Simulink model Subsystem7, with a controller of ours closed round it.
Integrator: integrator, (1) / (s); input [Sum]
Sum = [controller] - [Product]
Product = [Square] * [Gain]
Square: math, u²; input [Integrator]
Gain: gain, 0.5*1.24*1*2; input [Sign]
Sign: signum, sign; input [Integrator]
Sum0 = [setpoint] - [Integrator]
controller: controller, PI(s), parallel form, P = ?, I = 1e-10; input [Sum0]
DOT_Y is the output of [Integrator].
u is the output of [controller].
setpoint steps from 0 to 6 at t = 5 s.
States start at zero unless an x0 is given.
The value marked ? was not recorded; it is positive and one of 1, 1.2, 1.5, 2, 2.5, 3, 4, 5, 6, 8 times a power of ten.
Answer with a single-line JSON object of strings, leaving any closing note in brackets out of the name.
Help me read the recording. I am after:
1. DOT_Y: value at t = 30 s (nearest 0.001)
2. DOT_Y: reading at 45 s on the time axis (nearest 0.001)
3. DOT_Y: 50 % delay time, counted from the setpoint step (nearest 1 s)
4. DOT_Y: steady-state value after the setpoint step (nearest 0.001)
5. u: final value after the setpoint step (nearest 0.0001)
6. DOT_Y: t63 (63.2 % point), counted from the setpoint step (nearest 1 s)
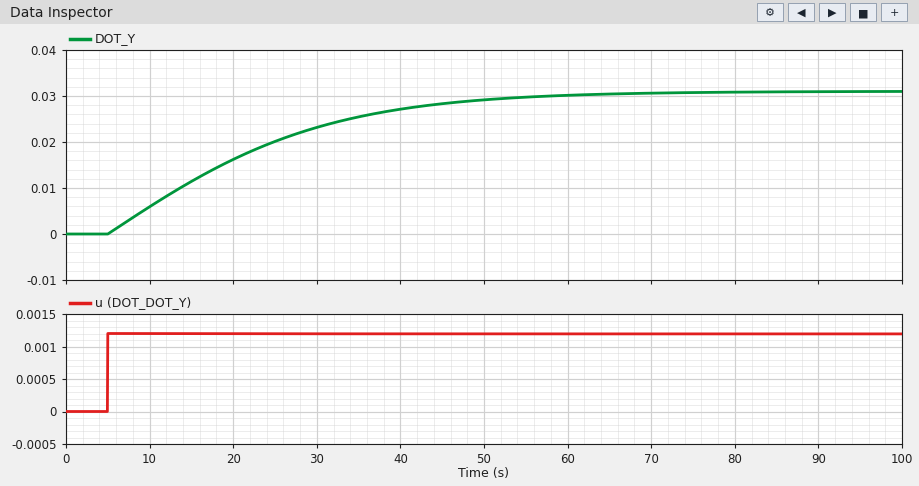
{"DOT_Y: value at t = 30 s": "0.023", "DOT_Y: reading at 45 s on the time axis": "0.028", "DOT_Y: 50 % delay time, counted from the setpoint step": "14 s", "DOT_Y: steady-state value after the setpoint step": "0.031", "u: final value after the setpoint step": "0.0012", "DOT_Y: t63 (63.2 % point), counted from the setpoint step": "19 s"}
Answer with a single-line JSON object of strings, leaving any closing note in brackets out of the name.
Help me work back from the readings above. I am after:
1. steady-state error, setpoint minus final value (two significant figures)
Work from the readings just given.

{"steady-state error, setpoint minus final value": "6.0"}
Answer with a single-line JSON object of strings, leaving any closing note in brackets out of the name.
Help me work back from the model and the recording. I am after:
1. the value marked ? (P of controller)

{"the value marked ?": "0.0002"}
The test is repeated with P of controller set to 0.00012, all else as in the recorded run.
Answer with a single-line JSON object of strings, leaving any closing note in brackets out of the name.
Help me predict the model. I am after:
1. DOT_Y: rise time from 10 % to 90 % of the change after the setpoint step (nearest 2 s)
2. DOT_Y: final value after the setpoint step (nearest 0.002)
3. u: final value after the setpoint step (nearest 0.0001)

{"DOT_Y: rise time from 10 % to 90 % of the change after the setpoint step": "46 s", "DOT_Y: final value after the setpoint step": "0.024", "u: final value after the setpoint step": "0.0007"}
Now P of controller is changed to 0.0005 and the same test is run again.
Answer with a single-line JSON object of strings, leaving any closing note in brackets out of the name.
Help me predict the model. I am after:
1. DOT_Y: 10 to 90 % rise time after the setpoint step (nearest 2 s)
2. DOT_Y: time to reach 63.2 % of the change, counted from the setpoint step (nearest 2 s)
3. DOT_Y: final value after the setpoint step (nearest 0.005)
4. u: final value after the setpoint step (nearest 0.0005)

{"DOT_Y: 10 to 90 % rise time after the setpoint step": "22 s", "DOT_Y: time to reach 63.2 % of the change, counted from the setpoint step": "12 s", "DOT_Y: final value after the setpoint step": "0.050", "u: final value after the setpoint step": "0.0030"}
